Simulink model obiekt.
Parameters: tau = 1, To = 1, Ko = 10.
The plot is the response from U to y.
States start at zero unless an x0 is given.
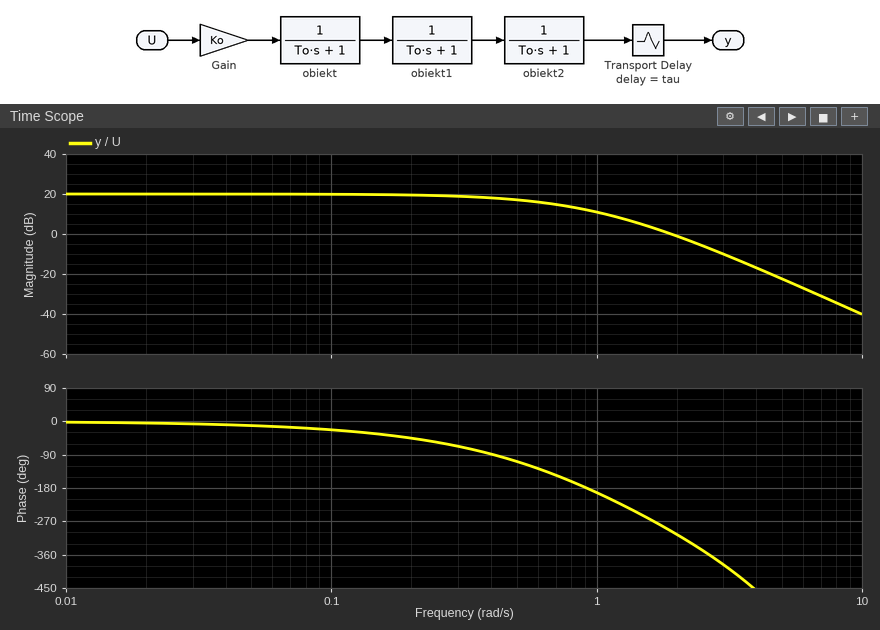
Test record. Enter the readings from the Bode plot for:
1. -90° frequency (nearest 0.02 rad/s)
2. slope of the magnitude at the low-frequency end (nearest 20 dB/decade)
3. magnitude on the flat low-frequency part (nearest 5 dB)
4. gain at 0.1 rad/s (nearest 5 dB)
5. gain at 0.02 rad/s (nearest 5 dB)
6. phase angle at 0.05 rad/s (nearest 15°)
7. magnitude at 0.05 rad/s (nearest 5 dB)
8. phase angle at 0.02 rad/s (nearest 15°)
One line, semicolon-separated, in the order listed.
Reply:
0.40 rad/s; 0 dB/decade; 20 dB; 20 dB; 20 dB; -15°; 20 dB; 0°
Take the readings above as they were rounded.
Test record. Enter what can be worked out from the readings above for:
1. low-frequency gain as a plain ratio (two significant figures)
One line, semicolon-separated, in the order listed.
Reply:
10
